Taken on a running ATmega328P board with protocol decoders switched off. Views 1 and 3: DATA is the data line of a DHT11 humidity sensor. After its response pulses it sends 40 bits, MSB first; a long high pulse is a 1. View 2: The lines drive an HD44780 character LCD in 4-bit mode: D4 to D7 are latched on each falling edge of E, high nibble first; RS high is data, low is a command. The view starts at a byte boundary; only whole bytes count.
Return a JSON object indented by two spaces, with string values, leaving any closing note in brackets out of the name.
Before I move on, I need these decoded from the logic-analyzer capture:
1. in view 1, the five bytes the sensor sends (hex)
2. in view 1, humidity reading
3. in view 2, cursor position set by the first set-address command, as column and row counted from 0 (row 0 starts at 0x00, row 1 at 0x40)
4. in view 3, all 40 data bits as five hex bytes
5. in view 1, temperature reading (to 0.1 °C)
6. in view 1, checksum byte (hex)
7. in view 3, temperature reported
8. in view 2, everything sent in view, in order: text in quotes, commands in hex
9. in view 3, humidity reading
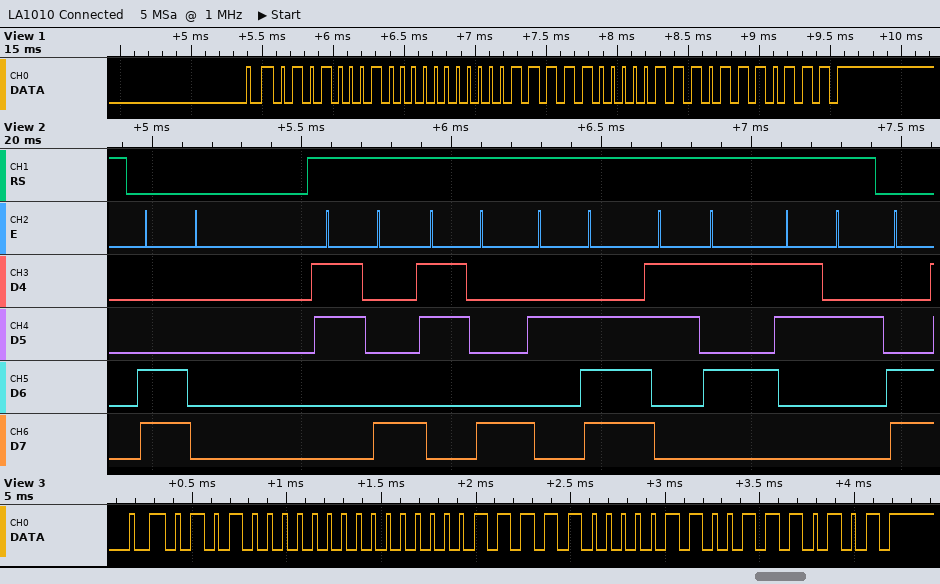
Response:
{
  "in view 1, the five bytes the sensor sends": "51 00 1F 07 77",
  "in view 1, humidity reading": "81 %",
  "in view 2, cursor position set by the first set-address command, as column and row counted from 0": "column 0, row 1",
  "in view 3, all 40 data bits as five hex bytes": "50 00 1F 06 75",
  "in view 1, temperature reading": "31.7 °C",
  "in view 1, checksum byte": "0x77",
  "in view 3, temperature reported": "31.6 °C",
  "in view 2, everything sent in view, in order: text in quotes, commands in hex": "0xC0 \"88.52\"",
  "in view 3, humidity reading": "80 %"
}
